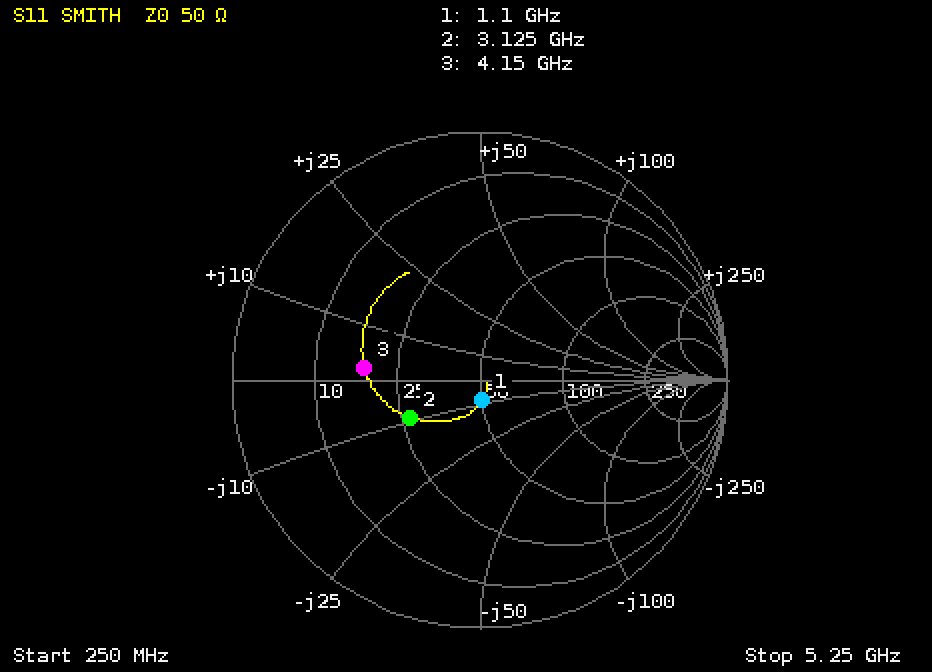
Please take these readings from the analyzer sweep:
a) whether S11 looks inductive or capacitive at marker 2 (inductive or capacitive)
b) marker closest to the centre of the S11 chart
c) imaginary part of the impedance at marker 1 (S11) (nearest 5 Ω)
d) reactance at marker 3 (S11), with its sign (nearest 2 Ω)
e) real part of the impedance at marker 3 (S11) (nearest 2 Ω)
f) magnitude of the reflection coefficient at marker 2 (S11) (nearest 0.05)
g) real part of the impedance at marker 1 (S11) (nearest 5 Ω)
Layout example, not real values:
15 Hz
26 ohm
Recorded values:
capacitive
marker 1
-10 Ω
+2 Ω
18 Ω
0.30
50 Ω
